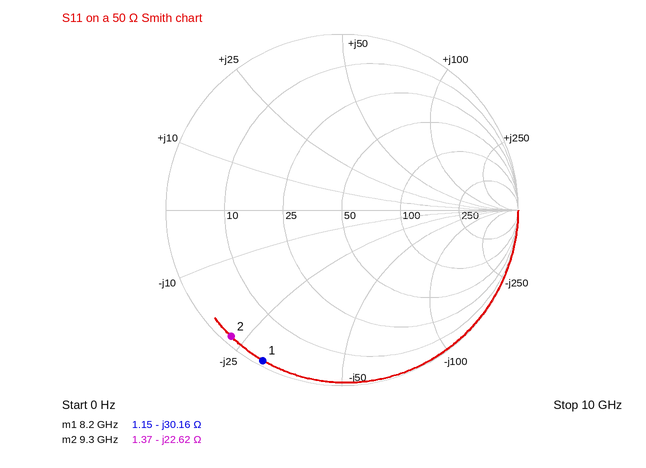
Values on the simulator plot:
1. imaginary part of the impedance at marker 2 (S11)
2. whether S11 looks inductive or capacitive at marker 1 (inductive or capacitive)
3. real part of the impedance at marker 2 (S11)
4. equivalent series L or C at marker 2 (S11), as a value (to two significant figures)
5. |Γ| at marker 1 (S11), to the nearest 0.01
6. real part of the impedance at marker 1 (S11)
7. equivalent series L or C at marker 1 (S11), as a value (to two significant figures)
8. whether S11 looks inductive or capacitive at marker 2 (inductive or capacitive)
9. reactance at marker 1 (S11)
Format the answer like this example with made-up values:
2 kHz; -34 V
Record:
-22.62 Ω; capacitive; 1.37 Ω; 760 fF; 0.97; 1.15 Ω; 640 fF; capacitive; -30.16 Ω
